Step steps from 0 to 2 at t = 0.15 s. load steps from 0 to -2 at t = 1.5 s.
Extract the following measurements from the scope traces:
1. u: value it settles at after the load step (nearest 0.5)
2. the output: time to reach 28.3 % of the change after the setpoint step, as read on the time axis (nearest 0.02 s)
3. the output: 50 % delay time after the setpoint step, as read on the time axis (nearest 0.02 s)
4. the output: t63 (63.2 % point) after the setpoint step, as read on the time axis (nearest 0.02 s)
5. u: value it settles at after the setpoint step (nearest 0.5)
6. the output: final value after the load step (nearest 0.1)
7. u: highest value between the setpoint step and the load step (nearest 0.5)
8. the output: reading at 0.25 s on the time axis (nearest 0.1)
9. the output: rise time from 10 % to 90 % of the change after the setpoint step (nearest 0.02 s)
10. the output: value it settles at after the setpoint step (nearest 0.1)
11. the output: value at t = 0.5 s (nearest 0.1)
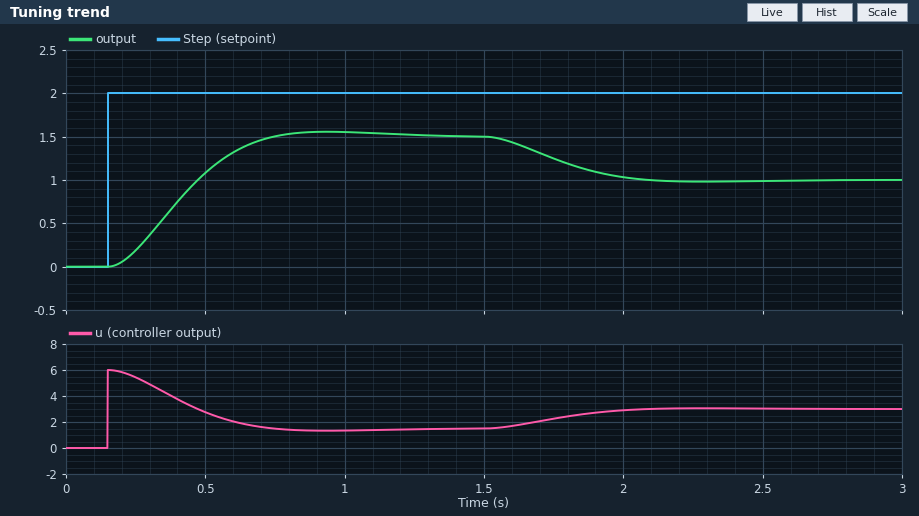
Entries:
3.0
0.32 s
0.40 s
0.46 s
1.5
1.0
6.0
0.2
0.38 s
1.5
1.1
